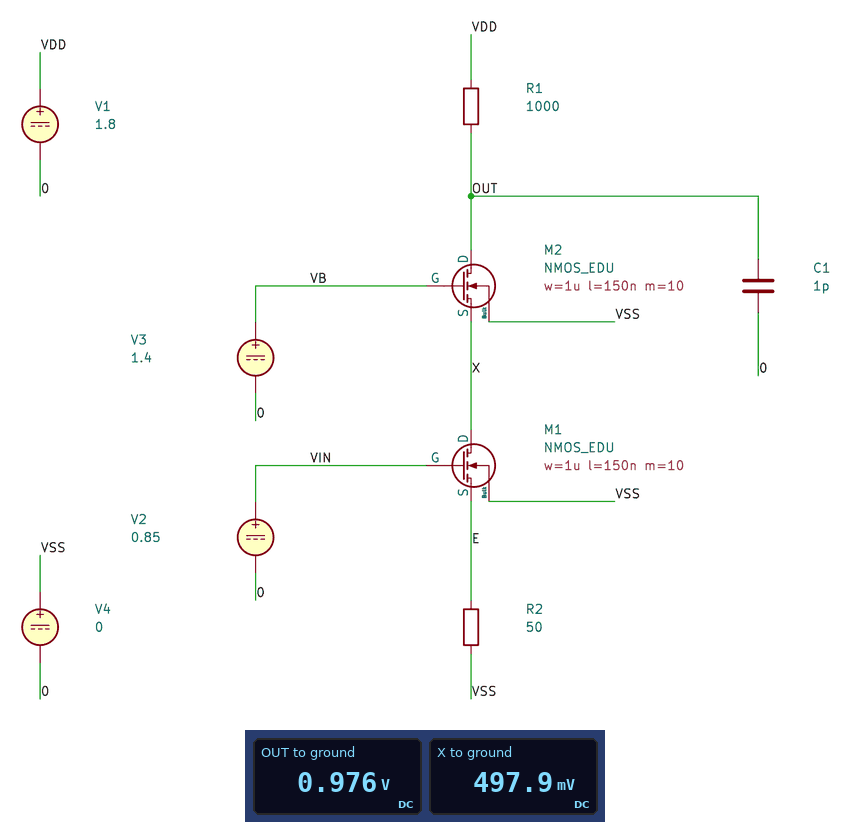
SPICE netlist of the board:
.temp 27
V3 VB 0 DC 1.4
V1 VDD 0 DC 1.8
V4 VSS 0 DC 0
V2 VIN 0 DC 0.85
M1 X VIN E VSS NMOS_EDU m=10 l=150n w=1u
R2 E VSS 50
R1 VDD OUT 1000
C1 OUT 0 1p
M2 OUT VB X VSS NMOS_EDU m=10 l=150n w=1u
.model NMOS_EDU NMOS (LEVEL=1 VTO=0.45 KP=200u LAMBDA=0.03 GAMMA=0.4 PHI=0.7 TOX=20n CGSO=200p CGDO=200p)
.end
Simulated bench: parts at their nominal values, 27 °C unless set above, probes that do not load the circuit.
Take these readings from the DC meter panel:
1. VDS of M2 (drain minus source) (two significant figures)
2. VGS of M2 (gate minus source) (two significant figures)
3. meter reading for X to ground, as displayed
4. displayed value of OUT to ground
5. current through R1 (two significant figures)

480 mV
900 mV
497.9 mV
0.976 V
820 µA
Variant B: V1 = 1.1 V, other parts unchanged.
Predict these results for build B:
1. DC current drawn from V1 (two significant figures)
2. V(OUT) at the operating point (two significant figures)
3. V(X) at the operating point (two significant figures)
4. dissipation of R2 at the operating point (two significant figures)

740 µA
360 mV
270 mV
27 µW
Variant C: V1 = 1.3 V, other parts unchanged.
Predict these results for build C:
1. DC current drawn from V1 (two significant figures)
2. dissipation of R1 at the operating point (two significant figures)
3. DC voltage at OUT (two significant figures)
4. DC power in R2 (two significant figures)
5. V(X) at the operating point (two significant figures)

810 µA
660 µW
490 mV
33 µW
350 mV
